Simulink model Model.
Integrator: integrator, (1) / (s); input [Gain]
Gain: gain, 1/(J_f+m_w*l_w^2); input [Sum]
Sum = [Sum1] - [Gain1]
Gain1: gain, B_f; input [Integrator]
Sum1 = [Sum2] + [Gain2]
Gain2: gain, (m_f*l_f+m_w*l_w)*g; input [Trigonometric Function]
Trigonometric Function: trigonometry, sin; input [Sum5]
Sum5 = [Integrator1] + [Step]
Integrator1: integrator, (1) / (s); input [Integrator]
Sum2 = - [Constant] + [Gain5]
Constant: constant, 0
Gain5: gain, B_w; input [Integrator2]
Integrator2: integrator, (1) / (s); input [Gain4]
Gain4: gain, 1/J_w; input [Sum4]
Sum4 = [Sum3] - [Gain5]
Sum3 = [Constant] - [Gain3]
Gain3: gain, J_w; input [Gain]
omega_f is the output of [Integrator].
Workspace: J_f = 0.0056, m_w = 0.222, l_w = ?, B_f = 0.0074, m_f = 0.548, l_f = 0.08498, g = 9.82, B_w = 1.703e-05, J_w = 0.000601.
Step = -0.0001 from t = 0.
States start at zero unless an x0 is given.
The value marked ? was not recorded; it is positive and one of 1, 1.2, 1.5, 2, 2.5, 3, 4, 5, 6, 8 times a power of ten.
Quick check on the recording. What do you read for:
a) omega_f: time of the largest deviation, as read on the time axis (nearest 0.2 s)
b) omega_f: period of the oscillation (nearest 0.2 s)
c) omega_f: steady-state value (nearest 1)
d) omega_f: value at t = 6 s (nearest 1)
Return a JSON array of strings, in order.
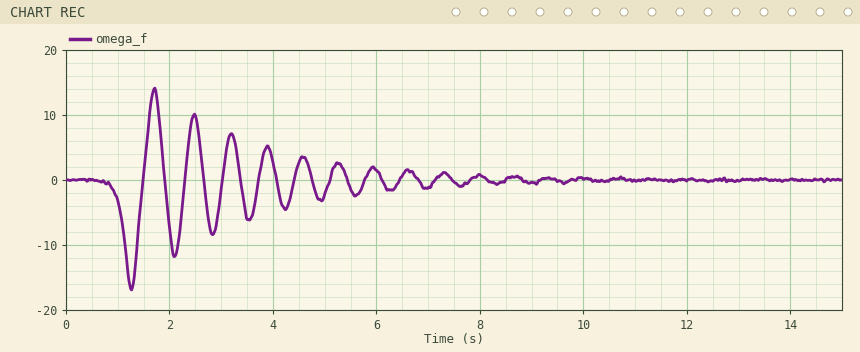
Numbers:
["1.2 s", "0.8 s", "0", "2"]
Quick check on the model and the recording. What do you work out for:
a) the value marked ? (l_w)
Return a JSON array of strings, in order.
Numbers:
["0.1"]
